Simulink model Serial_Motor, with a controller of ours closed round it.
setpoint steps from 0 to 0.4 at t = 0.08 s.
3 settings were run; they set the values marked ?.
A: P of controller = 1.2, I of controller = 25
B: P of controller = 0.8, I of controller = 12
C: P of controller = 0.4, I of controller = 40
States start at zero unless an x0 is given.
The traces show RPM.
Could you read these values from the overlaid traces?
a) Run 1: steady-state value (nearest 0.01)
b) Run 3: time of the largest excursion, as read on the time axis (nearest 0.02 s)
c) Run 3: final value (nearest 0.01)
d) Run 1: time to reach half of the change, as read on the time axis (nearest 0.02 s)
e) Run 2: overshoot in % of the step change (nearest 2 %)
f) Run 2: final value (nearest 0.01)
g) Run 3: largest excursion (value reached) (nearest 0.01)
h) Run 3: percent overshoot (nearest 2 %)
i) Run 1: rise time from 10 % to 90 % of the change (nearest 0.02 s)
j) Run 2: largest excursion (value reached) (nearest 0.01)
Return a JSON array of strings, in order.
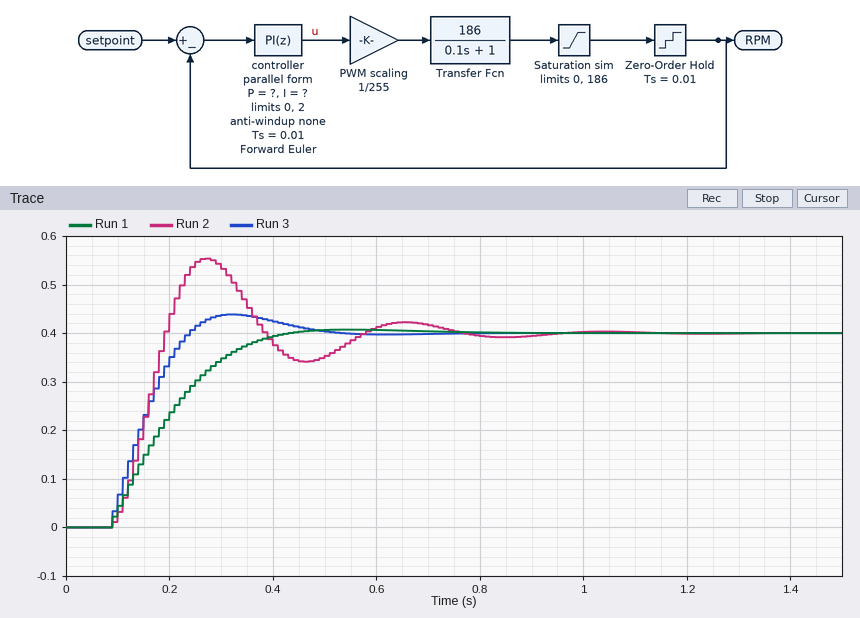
["0.40", "0.32 s", "0.40", "0.18 s", "38 %", "0.40", "0.44", "10 %", "0.22 s", "0.55"]
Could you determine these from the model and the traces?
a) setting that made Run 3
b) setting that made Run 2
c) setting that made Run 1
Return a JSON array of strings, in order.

["A", "C", "B"]
